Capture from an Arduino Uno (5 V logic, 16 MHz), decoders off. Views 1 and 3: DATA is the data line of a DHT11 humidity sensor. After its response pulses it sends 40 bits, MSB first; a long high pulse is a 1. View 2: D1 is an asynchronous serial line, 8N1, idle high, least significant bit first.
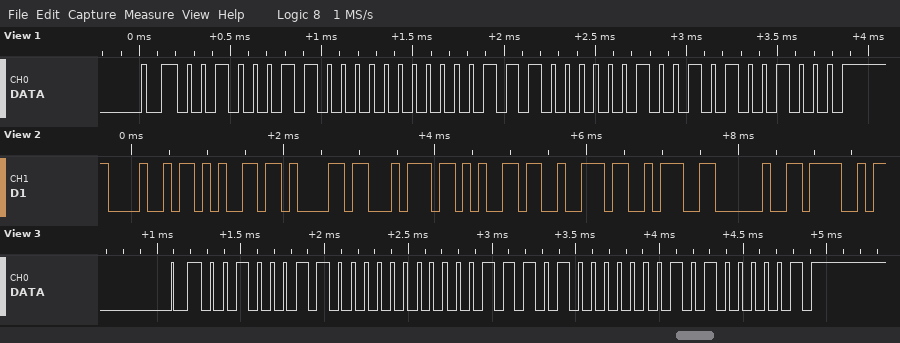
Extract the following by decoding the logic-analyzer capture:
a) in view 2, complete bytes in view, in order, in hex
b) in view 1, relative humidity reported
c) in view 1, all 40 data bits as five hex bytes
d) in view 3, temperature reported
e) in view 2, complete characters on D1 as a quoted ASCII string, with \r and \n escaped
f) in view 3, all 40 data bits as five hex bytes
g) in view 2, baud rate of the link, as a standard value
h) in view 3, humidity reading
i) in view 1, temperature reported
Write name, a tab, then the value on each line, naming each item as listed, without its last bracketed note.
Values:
in view 2, complete bytes in view, in order, in hex	0x48 0x65 0x61 0x74 0x65 0x72 0x3A 0x20 0x4F
in view 1, relative humidity reported	35 %
in view 1, all 40 data bits as five hex bytes	23 00 1C 09 48
in view 3, temperature reported	29.1 °C
in view 2, complete characters on D1 as a quoted ASCII string, with \r and \n escaped	"Heater: O"
in view 3, all 40 data bits as five hex bytes	23 00 1D 01 41
in view 2, baud rate of the link, as a standard value	9600 baud
in view 3, humidity reading	35 %
in view 1, temperature reported	28.9 °C
